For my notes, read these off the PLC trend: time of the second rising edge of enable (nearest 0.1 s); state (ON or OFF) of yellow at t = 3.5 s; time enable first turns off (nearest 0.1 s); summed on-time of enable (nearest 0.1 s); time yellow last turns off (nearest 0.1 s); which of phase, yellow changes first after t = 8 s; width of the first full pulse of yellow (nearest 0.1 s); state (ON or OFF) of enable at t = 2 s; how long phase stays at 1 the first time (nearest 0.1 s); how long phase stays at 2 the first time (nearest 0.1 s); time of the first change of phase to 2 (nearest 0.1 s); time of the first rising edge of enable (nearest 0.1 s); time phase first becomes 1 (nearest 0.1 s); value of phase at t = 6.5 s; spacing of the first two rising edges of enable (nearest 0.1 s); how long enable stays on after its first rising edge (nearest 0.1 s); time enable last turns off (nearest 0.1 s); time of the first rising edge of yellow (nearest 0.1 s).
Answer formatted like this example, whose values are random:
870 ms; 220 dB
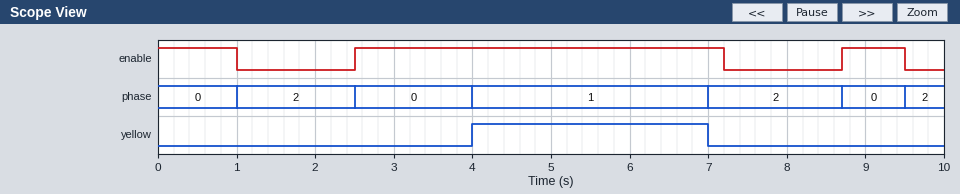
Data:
8.7 s; OFF; 1.0 s; 6.5 s; 7.0 s; phase; 3.0 s; OFF; 3.0 s; 1.5 s; 1.0 s; 2.5 s; 4.0 s; 1; 6.2 s; 4.7 s; 9.5 s; 4.0 s
